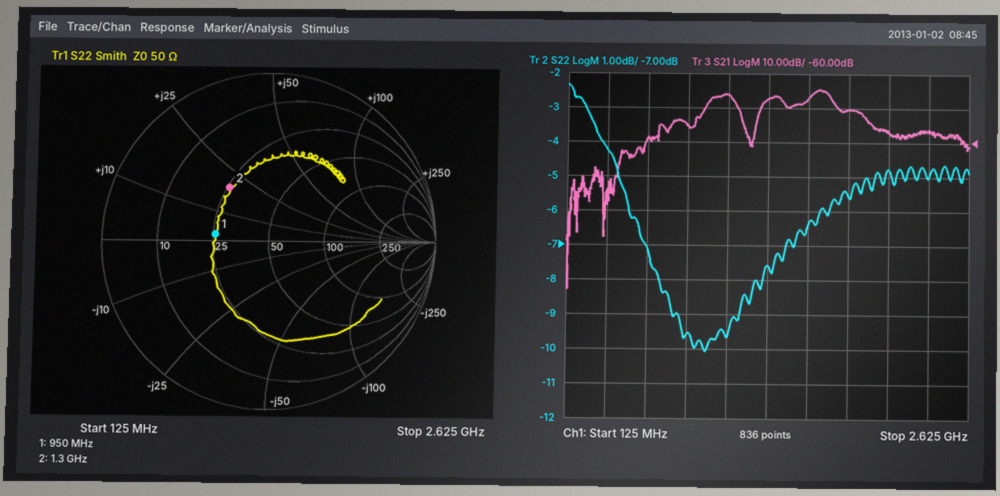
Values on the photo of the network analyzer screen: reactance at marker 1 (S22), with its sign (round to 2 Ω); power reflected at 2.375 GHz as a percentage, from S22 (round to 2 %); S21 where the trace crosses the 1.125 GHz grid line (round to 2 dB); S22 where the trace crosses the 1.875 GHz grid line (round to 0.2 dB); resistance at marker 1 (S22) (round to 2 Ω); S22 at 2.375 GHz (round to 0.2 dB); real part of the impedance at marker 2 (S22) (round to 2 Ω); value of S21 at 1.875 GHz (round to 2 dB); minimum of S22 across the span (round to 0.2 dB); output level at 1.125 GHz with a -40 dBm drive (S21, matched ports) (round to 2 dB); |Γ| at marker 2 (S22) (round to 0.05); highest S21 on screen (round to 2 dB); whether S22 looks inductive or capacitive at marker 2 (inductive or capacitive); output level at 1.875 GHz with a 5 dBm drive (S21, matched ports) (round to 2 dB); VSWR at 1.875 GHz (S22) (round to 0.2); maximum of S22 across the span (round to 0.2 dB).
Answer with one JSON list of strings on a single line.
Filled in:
["+2 Ω", "32 %", "-46 dB", "-5.6 dB", "26 Ω", "-5.0 dB", "26 Ω", "-50 dB", "-10.0 dB", "-86 dBm", "0.40", "-44 dB", "inductive", "-46 dBm", "3.2", "-2.4 dB"]
